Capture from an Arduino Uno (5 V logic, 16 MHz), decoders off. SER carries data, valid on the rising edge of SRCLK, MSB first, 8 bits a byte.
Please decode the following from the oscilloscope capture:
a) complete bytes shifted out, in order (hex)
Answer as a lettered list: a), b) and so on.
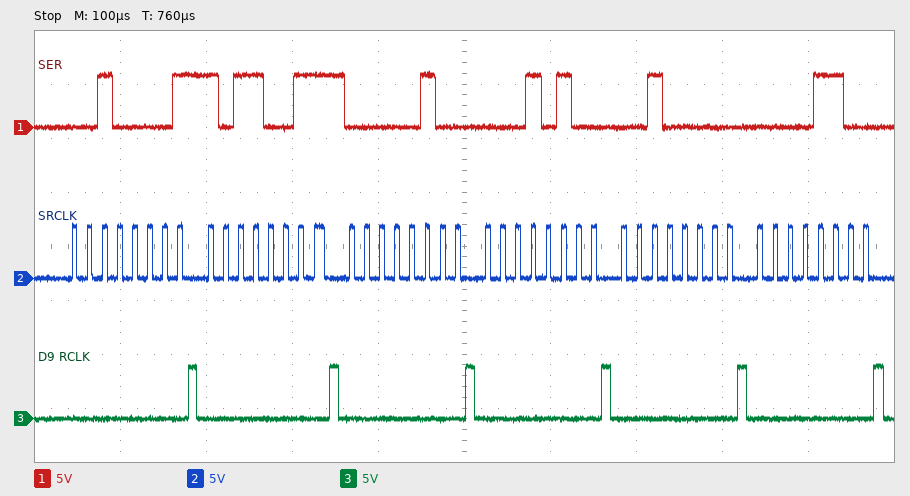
a) 21 B3 04 14 20 0C
